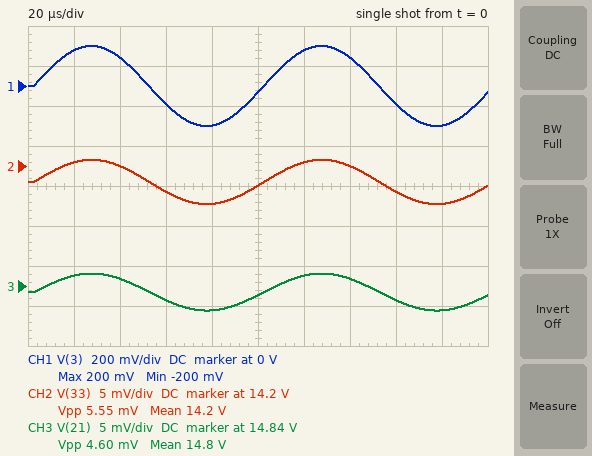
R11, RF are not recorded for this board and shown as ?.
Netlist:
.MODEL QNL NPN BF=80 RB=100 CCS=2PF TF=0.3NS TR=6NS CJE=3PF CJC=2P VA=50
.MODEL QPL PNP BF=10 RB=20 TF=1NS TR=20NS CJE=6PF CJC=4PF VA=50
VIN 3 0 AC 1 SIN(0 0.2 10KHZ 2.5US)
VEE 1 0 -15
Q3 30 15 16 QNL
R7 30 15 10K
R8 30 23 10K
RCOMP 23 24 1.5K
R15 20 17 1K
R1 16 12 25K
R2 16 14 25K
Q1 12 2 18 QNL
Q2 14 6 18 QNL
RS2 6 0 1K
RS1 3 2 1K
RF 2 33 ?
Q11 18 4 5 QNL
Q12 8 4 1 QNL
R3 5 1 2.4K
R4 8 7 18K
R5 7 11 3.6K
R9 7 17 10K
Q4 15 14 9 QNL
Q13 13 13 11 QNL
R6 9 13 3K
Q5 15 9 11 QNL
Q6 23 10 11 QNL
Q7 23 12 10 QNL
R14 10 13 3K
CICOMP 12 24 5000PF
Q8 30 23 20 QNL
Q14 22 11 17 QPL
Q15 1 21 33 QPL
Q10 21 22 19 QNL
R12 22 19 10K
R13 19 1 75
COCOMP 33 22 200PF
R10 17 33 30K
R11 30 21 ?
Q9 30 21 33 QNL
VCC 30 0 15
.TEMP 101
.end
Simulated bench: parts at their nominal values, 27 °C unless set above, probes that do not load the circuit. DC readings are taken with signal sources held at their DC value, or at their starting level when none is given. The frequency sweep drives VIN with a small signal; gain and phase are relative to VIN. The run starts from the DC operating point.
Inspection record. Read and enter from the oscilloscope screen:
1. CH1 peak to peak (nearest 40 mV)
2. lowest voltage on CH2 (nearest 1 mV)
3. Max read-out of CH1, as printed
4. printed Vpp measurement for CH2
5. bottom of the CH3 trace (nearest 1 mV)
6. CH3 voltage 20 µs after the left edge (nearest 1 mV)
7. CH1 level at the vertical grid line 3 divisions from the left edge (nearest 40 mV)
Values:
400 mV
14.190 V
200 mV
5.55 mV
14.832 V
14.836 V
-80 mV
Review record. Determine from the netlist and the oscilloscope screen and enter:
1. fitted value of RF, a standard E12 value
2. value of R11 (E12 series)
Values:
33 kΩ
33 kΩ
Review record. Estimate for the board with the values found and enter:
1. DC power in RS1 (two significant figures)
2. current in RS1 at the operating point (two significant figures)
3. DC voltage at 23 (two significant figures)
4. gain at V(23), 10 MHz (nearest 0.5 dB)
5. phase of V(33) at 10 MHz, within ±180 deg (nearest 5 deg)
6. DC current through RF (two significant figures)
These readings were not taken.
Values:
170 µW
420 µA
15 V
-25.5 dB
-15 deg
420 µA
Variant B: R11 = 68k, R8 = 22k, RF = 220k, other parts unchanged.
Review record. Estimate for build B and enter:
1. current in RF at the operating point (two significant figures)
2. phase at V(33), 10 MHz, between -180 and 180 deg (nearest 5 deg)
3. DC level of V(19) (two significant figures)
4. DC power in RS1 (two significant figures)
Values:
65 µA
-20 deg
-15 V
4.2 µW
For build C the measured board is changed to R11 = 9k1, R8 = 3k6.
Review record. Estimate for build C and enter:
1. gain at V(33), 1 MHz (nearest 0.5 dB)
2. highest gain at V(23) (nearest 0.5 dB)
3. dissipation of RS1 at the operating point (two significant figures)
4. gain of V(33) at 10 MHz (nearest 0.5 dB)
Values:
-45.0 dB
-26.5 dB
180 µW
-42.0 dB
